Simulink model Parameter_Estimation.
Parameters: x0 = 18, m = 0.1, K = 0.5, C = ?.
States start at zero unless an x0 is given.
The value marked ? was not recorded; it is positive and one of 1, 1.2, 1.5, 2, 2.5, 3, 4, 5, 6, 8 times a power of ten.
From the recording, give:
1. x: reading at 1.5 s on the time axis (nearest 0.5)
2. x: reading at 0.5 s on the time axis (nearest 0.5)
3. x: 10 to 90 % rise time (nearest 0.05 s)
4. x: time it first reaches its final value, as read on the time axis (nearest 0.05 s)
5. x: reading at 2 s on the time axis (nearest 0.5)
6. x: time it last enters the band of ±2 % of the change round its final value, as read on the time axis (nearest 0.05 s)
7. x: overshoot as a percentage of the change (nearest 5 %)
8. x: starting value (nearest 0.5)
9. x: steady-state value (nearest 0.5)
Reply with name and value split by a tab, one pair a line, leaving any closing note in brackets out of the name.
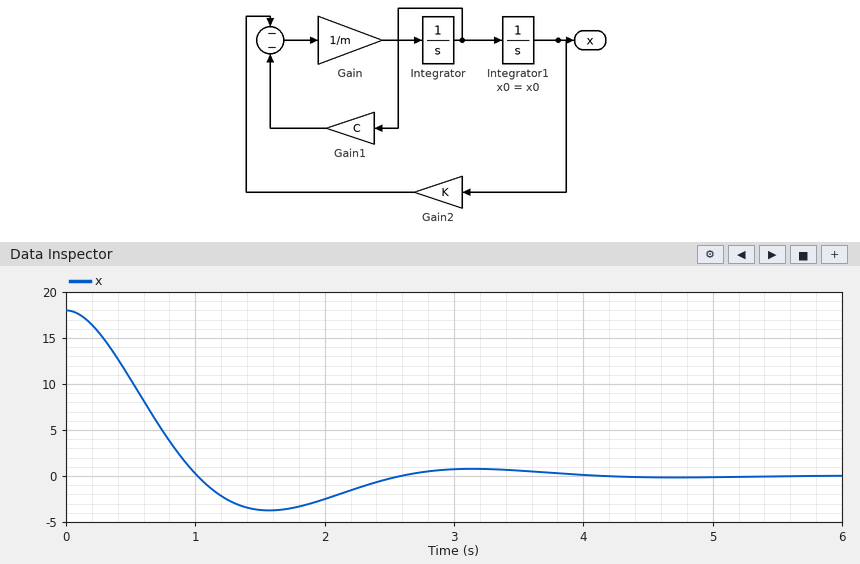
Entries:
x: reading at 1.5 s on the time axis	-3.5
x: reading at 0.5 s on the time axis	10.5
x: 10 to 90 % rise time	0.70 s
x: time it first reaches its final value, as read on the time axis	1.00 s
x: reading at 2 s on the time axis	-2.5
x: time it last enters the band of ±2 % of the change round its final value, as read on the time axis	3.75 s
x: overshoot as a percentage of the change	20 %
x: starting value	18.0
x: steady-state value	0.0
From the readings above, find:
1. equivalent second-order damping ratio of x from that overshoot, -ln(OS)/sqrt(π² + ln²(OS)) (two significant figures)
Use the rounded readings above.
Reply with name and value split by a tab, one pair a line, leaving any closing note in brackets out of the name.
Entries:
equivalent second-order damping ratio of x from that overshoot, -ln(OS)/sqrt(π² + ln²(OS))	0.46
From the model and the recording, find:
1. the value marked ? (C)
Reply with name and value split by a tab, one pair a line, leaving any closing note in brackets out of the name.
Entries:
the value marked ?	0.2
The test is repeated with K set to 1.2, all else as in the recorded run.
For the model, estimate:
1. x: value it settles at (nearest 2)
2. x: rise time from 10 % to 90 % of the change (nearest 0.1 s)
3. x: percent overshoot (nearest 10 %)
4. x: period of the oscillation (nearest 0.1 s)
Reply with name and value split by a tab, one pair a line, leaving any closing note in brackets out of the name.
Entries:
x: value it settles at	0
x: rise time from 10 % to 90 % of the change	0.4 s
x: percent overshoot	40 %
x: period of the oscillation	1.9 s
